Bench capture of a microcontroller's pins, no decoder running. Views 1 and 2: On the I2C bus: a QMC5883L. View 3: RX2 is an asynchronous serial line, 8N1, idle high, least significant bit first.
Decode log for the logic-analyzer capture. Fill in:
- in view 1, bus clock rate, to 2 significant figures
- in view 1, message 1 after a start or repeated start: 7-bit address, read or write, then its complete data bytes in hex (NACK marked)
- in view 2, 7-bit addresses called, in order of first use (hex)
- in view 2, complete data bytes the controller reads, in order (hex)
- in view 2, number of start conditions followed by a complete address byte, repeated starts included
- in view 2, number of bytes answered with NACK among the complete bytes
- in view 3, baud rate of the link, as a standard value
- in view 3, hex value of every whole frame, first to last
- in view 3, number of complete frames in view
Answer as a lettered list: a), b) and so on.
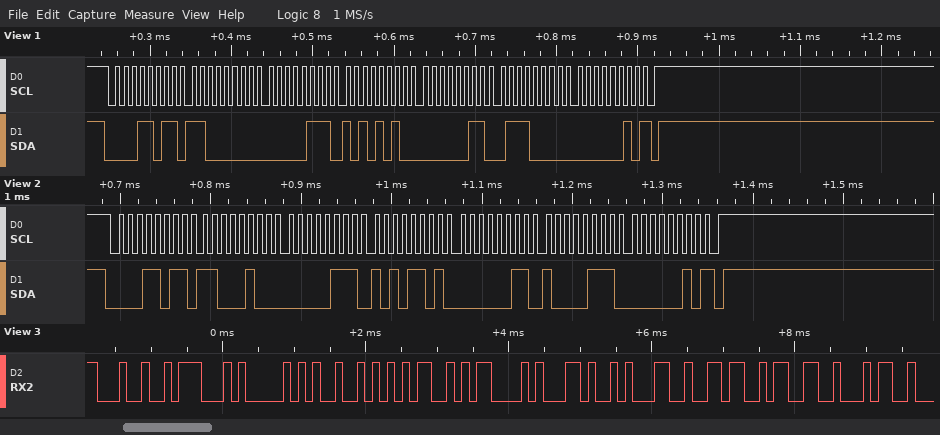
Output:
a) 100 kHz
b) 0x0D read: C0 07 AA 03 70 02 NACK
c) 0x0D
d) C4 07 AD 03 87 02
e) 1
f) 1
g) 9600 baud
h) 24 47 50 52 4D 43 2C 31 36 33 34
i) 11
